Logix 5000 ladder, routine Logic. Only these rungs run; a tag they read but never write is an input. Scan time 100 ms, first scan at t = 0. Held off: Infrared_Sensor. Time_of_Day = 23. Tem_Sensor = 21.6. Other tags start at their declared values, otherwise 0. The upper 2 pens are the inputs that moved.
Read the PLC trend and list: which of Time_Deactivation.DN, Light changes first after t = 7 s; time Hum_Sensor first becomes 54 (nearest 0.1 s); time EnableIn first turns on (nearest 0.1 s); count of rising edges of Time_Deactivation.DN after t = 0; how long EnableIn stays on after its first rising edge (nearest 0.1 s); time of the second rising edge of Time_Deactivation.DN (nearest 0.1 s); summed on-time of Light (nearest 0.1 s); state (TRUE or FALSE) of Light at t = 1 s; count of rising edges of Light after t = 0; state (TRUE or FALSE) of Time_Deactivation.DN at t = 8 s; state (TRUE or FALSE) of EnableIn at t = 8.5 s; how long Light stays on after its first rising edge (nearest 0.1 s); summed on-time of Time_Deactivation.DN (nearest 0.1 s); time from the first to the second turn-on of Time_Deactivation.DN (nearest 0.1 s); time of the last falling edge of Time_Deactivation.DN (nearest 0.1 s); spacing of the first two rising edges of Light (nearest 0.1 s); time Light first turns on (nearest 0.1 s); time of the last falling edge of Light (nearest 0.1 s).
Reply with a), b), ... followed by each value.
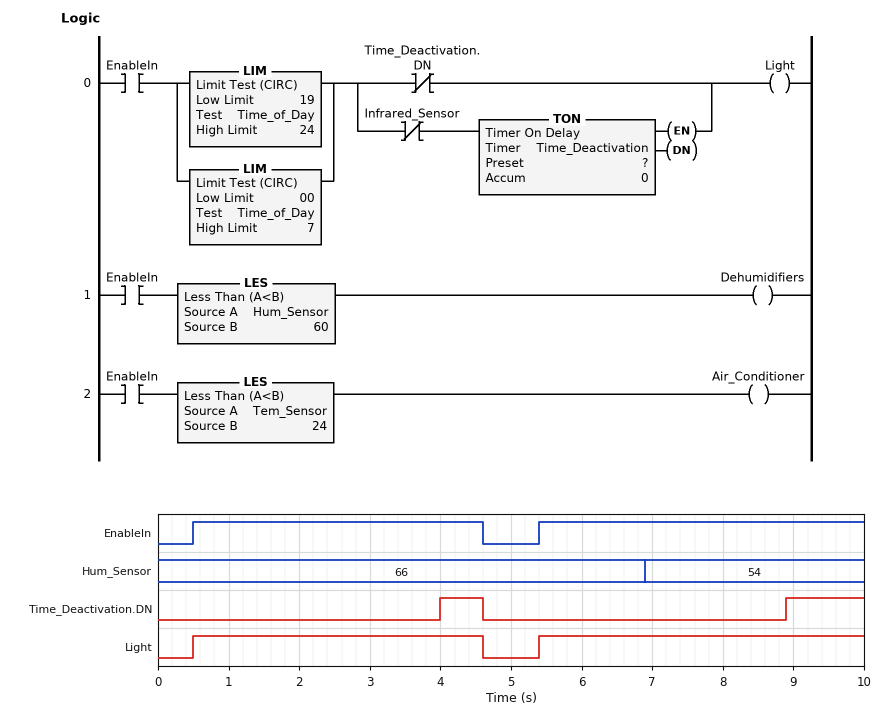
a) Time_Deactivation.DN
b) 6.9 s
c) 0.5 s
d) 2
e) 4.1 s
f) 8.9 s
g) 8.7 s
h) TRUE
i) 2
j) FALSE
k) TRUE
l) 4.1 s
m) 1.7 s
n) 4.9 s
o) 4.6 s
p) 4.9 s
q) 0.5 s
r) 4.6 s
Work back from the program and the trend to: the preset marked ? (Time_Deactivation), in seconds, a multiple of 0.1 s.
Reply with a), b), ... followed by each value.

a) 3.5 s
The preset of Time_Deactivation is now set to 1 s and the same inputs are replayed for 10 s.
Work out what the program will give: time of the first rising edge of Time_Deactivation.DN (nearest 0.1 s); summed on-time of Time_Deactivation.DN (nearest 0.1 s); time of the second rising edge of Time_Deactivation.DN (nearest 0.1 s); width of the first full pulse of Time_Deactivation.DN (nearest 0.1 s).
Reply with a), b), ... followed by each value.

a) 1.5 s
b) 6.7 s
c) 6.4 s
d) 3.1 s
